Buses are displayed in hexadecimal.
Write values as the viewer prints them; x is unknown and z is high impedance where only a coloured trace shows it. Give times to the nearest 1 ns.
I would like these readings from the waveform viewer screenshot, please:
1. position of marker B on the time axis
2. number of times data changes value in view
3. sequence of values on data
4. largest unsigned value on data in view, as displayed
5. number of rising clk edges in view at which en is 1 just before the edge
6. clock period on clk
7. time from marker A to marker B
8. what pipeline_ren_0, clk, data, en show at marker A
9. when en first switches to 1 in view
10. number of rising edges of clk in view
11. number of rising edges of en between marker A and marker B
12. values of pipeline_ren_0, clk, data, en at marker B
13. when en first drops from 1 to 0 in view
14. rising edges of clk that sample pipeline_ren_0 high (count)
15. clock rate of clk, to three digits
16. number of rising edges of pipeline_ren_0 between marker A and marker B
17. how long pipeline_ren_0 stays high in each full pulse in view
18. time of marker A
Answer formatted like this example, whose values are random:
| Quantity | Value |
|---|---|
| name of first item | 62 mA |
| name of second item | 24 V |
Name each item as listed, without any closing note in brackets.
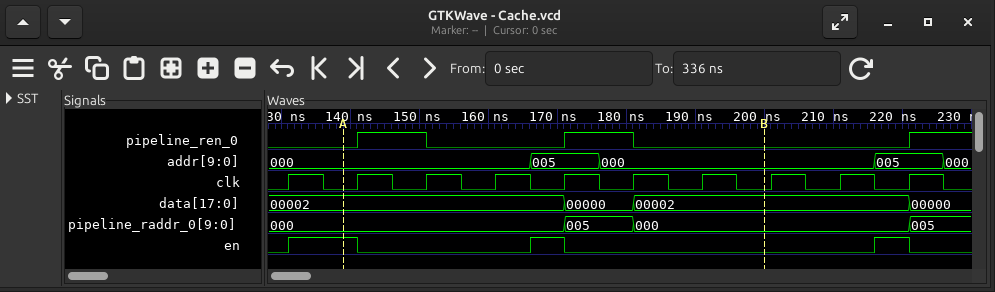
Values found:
| Quantity | Value |
|---|---|
| position of marker B on the time axis | 200 ns |
| number of times data changes value in view | 3 |
| sequence of values on data | 00002, 00000, 00002, 00000 |
| largest unsigned value on data in view, as displayed | 00002 |
| number of rising clk edges in view at which en is 1 just before the edge | 3 |
| clock period on clk | 10 ns |
| time from marker A to marker B | 61 ns |
| what pipeline_ren_0, clk, data, en show at marker A | pipeline_ren_0=0, clk=0, data=00002, en=1 |
| when en first switches to 1 in view | 131 ns |
| number of rising edges of clk in view | 10 |
| number of rising edges of en between marker A and marker B | 1 |
| values of pipeline_ren_0, clk, data, en at marker B | pipeline_ren_0=0, clk=0, data=00002, en=0 |
| when en first drops from 1 to 0 in view | 141 ns |
| rising edges of clk that sample pipeline_ren_0 high | 2 |
| clock rate of clk, to three digits | 100 MHz |
| number of rising edges of pipeline_ren_0 between marker A and marker B | 2 |
| how long pipeline_ren_0 stays high in each full pulse in view | 10 ns, 10 ns |
| time of marker A | 139 ns |
